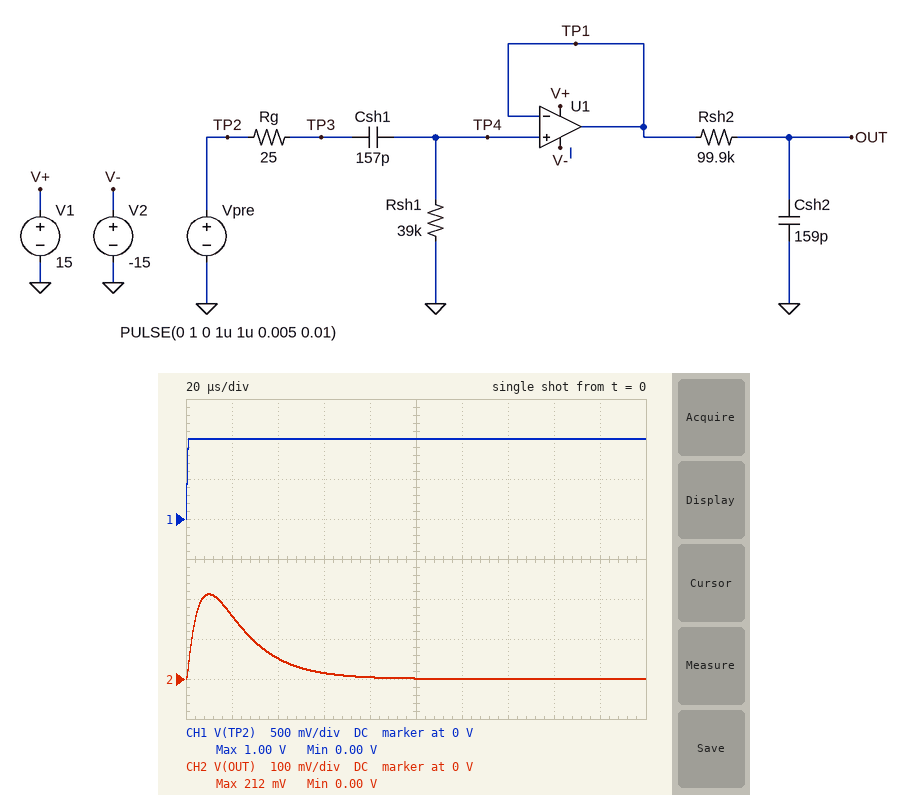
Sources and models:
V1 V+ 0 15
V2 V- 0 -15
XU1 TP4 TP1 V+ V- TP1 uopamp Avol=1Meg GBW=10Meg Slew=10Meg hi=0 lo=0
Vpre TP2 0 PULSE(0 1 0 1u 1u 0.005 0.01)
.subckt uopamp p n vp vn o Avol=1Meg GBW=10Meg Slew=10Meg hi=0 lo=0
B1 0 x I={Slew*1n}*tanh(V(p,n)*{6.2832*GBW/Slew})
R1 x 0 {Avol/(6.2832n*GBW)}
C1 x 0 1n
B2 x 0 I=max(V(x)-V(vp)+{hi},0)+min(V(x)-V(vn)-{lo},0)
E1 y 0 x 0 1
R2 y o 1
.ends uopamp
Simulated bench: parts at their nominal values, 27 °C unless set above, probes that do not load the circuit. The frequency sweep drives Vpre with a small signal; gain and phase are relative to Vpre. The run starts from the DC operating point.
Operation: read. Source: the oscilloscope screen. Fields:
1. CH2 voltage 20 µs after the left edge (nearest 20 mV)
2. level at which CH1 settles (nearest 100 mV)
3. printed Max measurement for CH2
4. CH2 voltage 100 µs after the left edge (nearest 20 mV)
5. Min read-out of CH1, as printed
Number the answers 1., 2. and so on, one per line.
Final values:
1. 160 mV
2. 1.0 V
3. 212 mV
4. 0 V
5. 0.00 V
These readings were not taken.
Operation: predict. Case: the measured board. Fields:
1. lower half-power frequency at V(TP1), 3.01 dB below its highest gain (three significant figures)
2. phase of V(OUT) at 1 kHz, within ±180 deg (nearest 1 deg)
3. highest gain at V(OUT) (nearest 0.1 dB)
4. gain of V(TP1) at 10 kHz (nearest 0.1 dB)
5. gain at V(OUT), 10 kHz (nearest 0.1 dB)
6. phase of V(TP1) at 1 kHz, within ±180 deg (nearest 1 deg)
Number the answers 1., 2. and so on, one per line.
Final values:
1. 25.8 kHz
2. 82 deg
3. -11.1 dB
4. -8.9 dB
5. -11.9 dB
6. 88 deg
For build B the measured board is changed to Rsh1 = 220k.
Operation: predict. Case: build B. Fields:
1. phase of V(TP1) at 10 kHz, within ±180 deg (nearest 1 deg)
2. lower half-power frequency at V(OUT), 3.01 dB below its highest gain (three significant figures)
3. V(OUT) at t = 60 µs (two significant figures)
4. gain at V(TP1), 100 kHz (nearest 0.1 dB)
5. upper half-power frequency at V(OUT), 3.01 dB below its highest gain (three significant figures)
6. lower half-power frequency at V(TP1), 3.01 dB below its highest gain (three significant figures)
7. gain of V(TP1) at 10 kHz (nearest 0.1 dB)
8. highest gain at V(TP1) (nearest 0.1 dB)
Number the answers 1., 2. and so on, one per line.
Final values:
1. 25 deg
2. 2.67 kHz
3. 290 mV
4. 0 dB
5. 17.3 kHz
6. 4.60 kHz
7. -0.8 dB
8. 0 dB
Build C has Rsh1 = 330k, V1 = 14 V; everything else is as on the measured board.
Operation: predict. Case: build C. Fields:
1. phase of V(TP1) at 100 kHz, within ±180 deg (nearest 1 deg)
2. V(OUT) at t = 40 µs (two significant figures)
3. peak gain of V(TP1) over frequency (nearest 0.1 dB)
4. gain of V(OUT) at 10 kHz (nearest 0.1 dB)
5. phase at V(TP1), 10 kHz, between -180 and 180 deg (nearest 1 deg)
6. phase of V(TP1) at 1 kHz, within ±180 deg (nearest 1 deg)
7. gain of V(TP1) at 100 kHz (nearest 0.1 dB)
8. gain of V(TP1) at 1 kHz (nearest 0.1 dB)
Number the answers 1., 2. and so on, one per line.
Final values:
1. 1 deg
2. 550 mV
3. 0 dB
4. -3.4 dB
5. 17 deg
6. 72 deg
7. 0 dB
8. -10.2 dB
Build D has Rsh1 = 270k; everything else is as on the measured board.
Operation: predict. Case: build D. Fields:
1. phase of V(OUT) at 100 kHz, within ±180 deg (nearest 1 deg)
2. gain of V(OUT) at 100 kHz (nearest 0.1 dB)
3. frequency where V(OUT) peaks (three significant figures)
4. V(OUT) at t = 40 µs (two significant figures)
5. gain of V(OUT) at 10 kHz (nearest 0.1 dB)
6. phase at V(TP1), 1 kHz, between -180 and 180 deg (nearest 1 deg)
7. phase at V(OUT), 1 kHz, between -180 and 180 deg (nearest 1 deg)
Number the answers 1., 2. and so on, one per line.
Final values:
1. -83 deg
2. -20.0 dB
3. 6.13 kHz
4. 500 mV
5. -3.6 dB
6. 75 deg
7. 69 deg
